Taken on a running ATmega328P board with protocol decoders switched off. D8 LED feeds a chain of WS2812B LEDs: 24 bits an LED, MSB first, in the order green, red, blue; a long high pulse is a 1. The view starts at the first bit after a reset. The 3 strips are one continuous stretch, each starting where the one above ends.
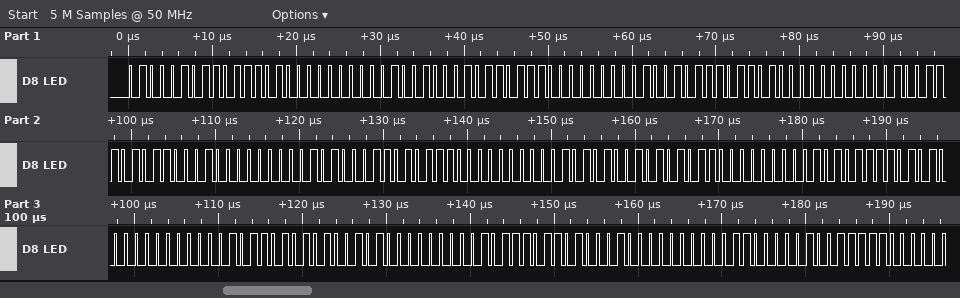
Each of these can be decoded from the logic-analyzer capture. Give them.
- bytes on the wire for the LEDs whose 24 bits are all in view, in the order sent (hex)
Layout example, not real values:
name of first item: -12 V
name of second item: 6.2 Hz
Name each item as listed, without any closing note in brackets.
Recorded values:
bytes on the wire for the LEDs whose 24 bits are all in view, in the order sent: 45 BA 00 48 B7 00 4B B4 00 4E B1 00 51 AE 00 54 AB 00 57 A8 00 5A A5 00 5D A2 00
